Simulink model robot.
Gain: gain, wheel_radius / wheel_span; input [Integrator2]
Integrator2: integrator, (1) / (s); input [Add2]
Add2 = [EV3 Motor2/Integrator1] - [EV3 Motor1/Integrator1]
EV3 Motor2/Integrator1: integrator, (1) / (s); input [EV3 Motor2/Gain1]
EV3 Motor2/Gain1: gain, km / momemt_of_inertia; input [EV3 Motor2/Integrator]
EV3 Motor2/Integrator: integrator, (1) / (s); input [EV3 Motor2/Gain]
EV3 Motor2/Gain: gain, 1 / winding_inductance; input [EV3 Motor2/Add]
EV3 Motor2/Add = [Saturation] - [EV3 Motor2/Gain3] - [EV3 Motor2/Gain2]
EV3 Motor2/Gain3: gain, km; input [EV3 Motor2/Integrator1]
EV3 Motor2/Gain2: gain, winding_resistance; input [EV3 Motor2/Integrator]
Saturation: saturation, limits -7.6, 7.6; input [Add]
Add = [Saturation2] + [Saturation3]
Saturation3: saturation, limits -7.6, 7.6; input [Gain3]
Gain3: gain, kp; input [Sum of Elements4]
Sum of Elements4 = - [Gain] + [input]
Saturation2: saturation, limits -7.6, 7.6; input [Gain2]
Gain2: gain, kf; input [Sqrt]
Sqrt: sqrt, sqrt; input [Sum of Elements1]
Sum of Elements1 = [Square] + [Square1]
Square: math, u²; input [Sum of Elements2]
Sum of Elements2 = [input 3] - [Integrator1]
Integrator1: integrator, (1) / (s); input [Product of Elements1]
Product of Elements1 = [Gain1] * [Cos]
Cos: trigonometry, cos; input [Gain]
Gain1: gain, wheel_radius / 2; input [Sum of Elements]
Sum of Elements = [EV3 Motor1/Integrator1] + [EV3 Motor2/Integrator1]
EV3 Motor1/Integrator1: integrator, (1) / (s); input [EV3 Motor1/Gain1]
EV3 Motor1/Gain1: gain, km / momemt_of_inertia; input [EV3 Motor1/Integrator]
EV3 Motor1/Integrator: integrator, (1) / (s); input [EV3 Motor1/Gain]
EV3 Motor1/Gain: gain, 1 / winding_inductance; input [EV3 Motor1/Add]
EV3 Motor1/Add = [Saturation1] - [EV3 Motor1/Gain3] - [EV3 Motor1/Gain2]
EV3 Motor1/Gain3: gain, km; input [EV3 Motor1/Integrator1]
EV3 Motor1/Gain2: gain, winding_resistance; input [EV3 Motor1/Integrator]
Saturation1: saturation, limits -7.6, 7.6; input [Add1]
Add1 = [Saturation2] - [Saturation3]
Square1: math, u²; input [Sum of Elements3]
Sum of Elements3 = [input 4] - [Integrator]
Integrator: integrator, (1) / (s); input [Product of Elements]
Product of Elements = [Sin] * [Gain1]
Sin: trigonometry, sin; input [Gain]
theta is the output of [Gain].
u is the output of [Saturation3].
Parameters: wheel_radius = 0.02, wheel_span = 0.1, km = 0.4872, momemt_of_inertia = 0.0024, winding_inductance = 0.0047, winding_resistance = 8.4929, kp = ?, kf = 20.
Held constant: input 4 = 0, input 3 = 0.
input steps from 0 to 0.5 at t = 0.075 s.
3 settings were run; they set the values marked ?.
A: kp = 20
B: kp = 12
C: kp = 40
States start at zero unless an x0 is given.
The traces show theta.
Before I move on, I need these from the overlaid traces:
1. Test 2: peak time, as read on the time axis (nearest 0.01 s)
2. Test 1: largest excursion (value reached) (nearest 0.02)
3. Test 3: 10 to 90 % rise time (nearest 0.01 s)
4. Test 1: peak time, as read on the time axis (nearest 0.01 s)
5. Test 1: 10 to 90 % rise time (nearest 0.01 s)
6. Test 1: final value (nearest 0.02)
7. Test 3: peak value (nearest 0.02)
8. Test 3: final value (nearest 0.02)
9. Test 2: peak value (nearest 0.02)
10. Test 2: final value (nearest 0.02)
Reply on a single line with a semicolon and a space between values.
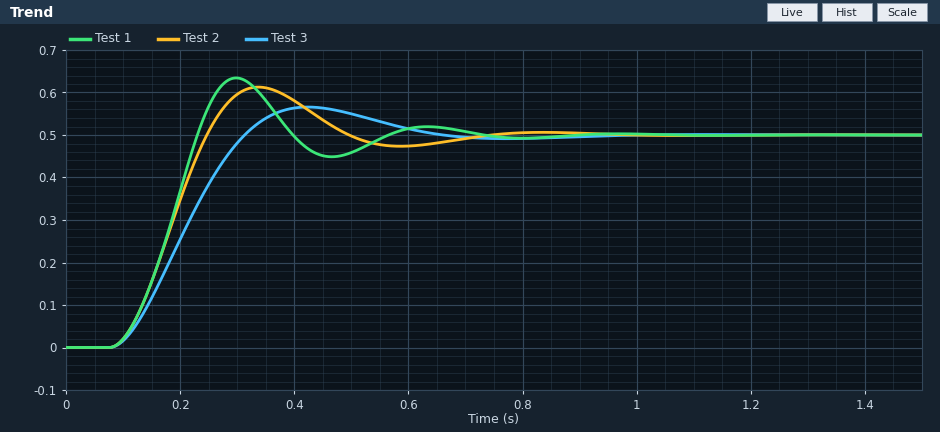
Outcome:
0.34 s; 0.64; 0.16 s; 0.30 s; 0.10 s; 0.50; 0.56; 0.50; 0.62; 0.50
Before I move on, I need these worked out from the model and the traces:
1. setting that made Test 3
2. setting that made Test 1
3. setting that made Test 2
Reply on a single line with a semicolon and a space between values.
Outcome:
B; C; A
